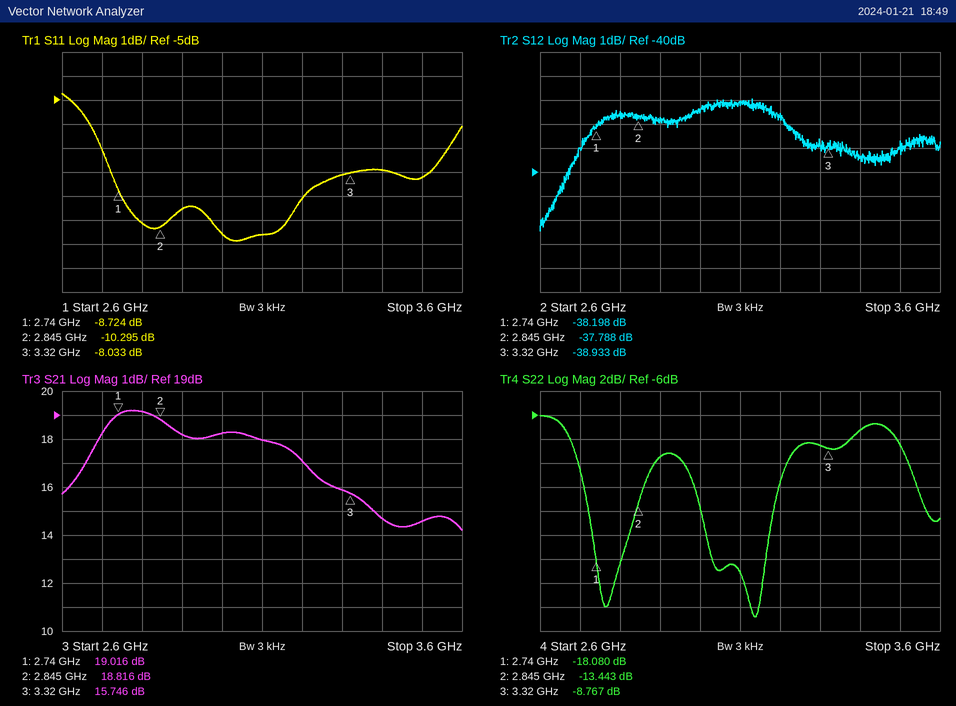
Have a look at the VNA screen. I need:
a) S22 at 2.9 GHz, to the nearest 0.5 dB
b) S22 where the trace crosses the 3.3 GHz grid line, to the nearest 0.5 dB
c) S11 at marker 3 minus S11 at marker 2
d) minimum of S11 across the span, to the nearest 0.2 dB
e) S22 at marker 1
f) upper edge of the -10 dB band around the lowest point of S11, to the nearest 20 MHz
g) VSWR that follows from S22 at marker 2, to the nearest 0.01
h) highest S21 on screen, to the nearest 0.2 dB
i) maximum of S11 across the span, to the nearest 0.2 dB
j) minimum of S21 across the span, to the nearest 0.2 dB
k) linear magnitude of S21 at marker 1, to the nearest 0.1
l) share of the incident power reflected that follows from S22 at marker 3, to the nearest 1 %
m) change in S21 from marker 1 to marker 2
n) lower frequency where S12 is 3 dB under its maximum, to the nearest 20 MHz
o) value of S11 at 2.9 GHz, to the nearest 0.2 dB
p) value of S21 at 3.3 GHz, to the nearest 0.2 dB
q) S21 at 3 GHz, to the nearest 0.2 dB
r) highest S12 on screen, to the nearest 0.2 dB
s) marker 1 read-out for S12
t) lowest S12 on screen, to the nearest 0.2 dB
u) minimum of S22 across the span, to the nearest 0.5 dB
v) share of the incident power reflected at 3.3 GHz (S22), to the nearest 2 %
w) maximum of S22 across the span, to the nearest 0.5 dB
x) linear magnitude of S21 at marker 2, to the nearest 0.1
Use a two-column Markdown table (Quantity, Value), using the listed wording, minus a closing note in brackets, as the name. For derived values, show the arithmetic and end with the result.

| Quantity | Value |
|---|---|
| S22 at 2.9 GHz, to the nearest 0.5 dB | -9.5 dB |
| S22 where the trace crosses the 3.3 GHz grid line, to the nearest 0.5 dB | -8.5 dB |
| S11 at marker 3 minus S11 at marker 2 | -8.033 − (-10.295) = 2.262 dB |
| minimum of S11 across the span, to the nearest 0.2 dB | -10.8 dB |
| S22 at marker 1 | -18.080 dB |
| upper edge of the -10 dB band around the lowest point of S11, to the nearest 20 MHz | 3.16 GHz |
| VSWR that follows from S22 at marker 2, to the nearest 0.01 | (1 + 0.2127)/(1 − 0.2127) ≈ 1.54 |
| highest S21 on screen, to the nearest 0.2 dB | 19.2 dB |
| maximum of S11 across the span, to the nearest 0.2 dB | -4.8 dB |
| minimum of S21 across the span, to the nearest 0.2 dB | 14.2 dB |
| linear magnitude of S21 at marker 1, to the nearest 0.1 | 10^(19.016/20) ≈ 8.9 |
| share of the incident power reflected that follows from S22 at marker 3, to the nearest 1 % | 10^(-8.767/10) ≈ 13 % |
| change in S21 from marker 1 to marker 2 | 18.816 − (19.016) = -0.200 dB |
| lower frequency where S12 is 3 dB under its maximum, to the nearest 20 MHz | 2.68 GHz |
| value of S11 at 2.9 GHz, to the nearest 0.2 dB | -9.6 dB |
| value of S21 at 3.3 GHz, to the nearest 0.2 dB | 15.8 dB |
| S21 at 3 GHz, to the nearest 0.2 dB | 18.2 dB |
| highest S12 on screen, to the nearest 0.2 dB | -37.0 dB |
| marker 1 read-out for S12 | -38.198 dB |
| lowest S12 on screen, to the nearest 0.2 dB | -42.4 dB |
| minimum of S22 across the span, to the nearest 0.5 dB | -23.0 dB |
| share of the incident power reflected at 3.3 GHz (S22), to the nearest 2 % | 10^(-8.5/10) ≈ 14 % |
| maximum of S22 across the span, to the nearest 0.5 dB | -6.0 dB |
| linear magnitude of S21 at marker 2, to the nearest 0.1 | 10^(18.816/20) ≈ 8.7 |
